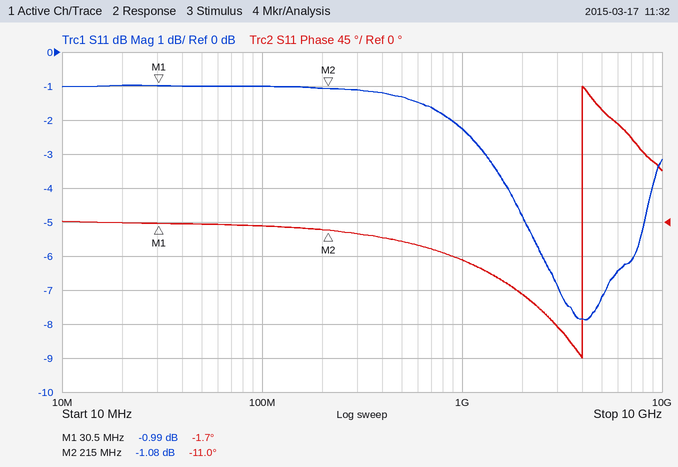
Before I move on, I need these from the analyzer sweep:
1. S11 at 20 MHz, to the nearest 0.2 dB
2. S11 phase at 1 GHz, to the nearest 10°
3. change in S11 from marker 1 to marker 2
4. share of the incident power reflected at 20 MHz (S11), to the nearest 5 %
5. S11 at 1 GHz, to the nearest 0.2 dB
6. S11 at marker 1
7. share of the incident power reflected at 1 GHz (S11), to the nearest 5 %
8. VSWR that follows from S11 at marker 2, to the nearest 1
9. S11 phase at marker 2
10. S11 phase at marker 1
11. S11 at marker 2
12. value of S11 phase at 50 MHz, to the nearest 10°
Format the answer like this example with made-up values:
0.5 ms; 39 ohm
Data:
-1.0 dB; -50°; -0.09 dB; 80 %; -2.2 dB; -0.99 dB; 60 %; 16; -11.0°; -1.7°; -1.08 dB; 0°
